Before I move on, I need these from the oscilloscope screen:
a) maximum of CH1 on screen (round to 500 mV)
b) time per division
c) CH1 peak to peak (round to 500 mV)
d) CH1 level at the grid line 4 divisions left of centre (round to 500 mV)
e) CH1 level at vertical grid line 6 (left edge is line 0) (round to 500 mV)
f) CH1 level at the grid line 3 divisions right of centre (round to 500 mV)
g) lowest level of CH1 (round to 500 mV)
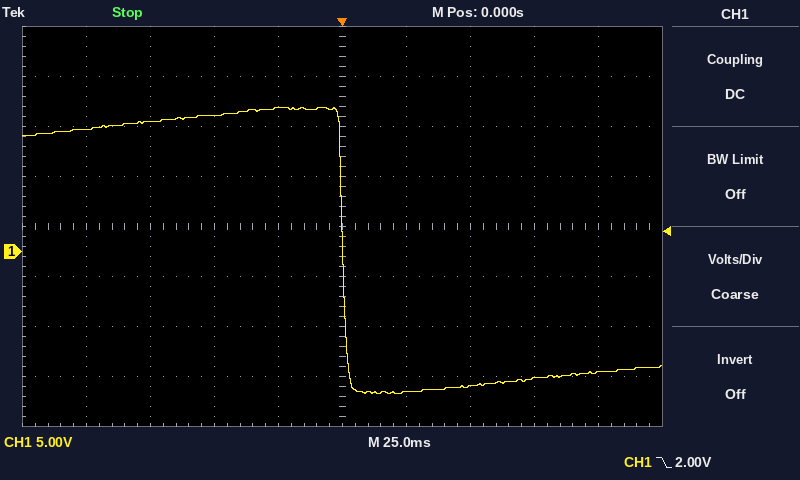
14.5 V
25 ms
28.5 V
12.0 V
-14.0 V
-12.5 V
-14.0 V
